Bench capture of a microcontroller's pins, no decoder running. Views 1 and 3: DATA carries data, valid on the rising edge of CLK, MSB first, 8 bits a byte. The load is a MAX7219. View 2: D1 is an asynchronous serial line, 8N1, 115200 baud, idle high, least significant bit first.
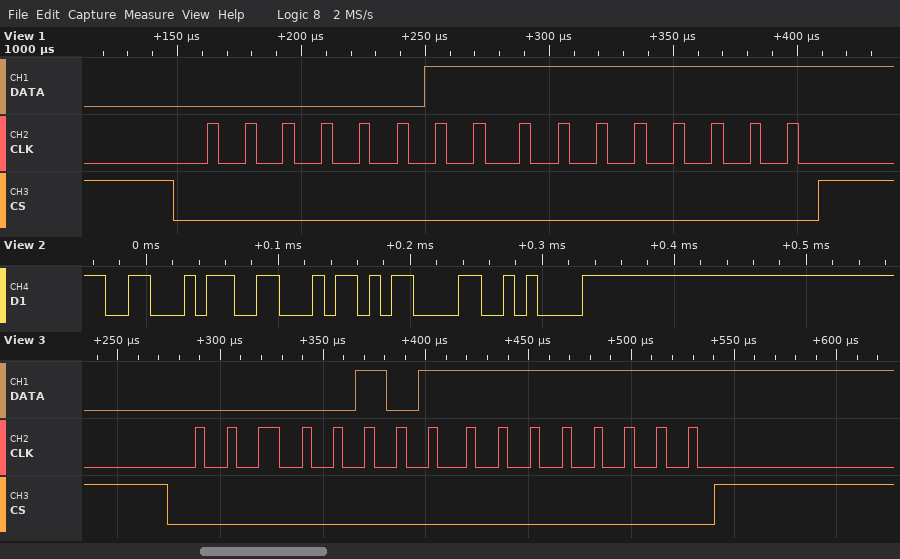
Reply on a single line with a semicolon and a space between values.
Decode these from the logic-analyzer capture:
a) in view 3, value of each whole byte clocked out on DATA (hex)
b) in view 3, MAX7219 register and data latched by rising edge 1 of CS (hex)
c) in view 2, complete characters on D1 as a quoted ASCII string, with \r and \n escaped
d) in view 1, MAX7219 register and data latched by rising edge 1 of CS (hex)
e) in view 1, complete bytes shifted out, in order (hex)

0x05 0xFF; register 0x5, data 0xFF; "FF\r\n"; register 0x3, data 0xFF; 03 FF
